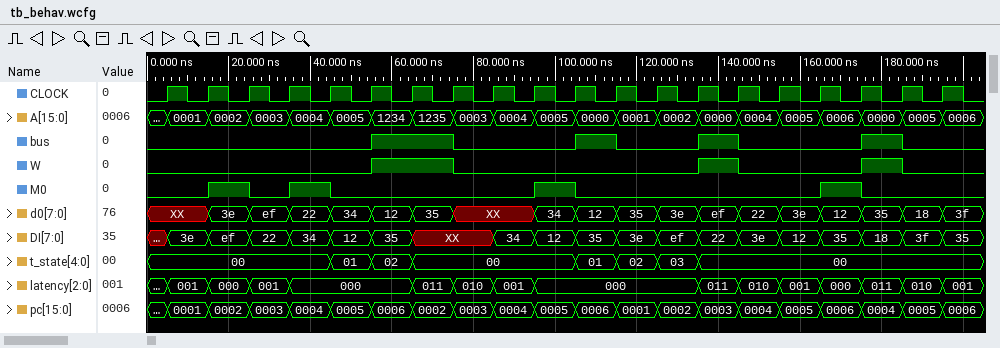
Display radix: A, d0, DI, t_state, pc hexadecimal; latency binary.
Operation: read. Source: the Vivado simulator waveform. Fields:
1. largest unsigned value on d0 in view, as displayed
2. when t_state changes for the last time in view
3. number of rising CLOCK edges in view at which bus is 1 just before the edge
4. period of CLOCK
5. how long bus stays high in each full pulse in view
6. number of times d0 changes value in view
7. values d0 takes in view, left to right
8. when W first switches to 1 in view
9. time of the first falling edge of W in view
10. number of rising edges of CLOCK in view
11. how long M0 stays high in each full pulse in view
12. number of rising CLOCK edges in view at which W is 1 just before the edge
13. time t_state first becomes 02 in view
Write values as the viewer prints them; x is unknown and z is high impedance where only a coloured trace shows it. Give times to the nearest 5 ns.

ef
135 ns
5
10 ns
20 ns, 10 ns, 10 ns, 10 ns
18
XX, 3e, ef, 22, 34, 12, 35, XX, 34, 12, 35, 3e, ef, 22, 3e, 12, 35, 18, 3f
55 ns
75 ns
20
10 ns, 10 ns, 10 ns, 10 ns
4
55 ns
